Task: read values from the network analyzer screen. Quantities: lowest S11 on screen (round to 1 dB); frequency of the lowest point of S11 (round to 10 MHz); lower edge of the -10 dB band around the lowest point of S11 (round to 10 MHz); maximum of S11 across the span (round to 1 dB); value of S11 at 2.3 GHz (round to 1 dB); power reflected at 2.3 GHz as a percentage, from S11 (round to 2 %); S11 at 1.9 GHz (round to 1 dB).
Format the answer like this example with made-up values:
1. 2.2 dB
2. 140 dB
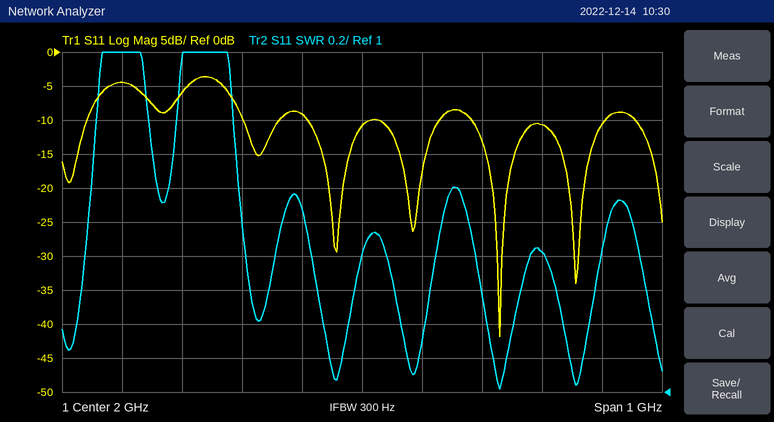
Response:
1. -42 dB
2. 2.23 GHz
3. 2.18 GHz
4. -4 dB
5. -11 dB
6. 8 %
7. -9 dB
